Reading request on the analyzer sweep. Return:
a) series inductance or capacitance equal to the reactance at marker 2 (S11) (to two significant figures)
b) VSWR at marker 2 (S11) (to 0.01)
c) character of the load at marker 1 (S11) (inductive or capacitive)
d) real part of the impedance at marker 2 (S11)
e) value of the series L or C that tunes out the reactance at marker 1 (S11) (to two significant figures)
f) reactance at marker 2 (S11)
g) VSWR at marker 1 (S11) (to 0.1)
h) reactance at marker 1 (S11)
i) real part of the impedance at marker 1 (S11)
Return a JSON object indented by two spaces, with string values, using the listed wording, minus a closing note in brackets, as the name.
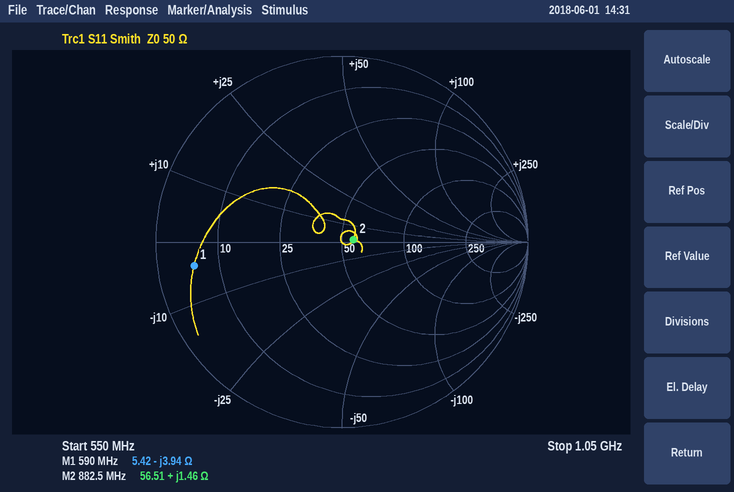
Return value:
{
  "series inductance or capacitance equal to the reactance at marker 2 (S11)": "260 pH",
  "VSWR at marker 2 (S11)": "1.13",
  "character of the load at marker 1 (S11)": "capacitive",
  "real part of the impedance at marker 2": "56.51 Ω",
  "value of the series L or C that tunes out the reactance at marker 1 (S11)": "1.1 nH",
  "reactance at marker 2": "+1.46 Ω",
  "VSWR at marker 1 (S11)": "9.3",
  "reactance at marker 1": "-3.94 Ω",
  "real part of the impedance at marker 1": "5.42 Ω"
}
